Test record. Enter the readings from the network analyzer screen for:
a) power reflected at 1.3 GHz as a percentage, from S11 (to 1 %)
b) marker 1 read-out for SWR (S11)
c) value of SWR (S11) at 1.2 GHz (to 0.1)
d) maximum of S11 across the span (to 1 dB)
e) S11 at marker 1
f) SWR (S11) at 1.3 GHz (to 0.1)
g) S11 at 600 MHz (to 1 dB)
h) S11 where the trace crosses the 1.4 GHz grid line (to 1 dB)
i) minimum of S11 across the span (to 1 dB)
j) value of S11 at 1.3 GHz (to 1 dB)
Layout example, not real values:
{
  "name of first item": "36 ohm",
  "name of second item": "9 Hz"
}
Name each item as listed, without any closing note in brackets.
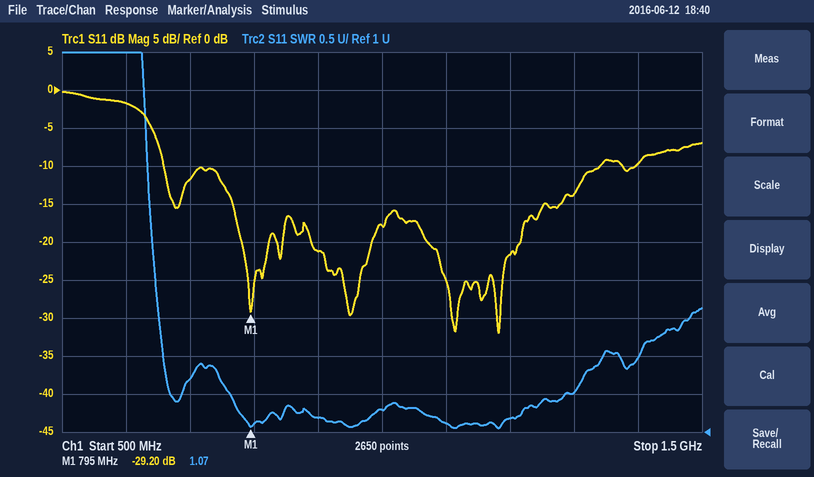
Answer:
{
  "power reflected at 1.3 GHz as a percentage, from S11": "4 %",
  "marker 1 read-out for SWR": "1.07",
  "value of SWR (S11) at 1.2 GHz": "1.2",
  "maximum of S11 across the span": "0 dB",
  "S11 at marker 1": "-29.20 dB",
  "SWR (S11) at 1.3 GHz": "1.5",
  "S11 at 600 MHz": "-2 dB",
  "S11 where the trace crosses the 1.4 GHz grid line": "-10 dB",
  "minimum of S11 across the span": "-32 dB",
  "value of S11 at 1.3 GHz": "-14 dB"
}
